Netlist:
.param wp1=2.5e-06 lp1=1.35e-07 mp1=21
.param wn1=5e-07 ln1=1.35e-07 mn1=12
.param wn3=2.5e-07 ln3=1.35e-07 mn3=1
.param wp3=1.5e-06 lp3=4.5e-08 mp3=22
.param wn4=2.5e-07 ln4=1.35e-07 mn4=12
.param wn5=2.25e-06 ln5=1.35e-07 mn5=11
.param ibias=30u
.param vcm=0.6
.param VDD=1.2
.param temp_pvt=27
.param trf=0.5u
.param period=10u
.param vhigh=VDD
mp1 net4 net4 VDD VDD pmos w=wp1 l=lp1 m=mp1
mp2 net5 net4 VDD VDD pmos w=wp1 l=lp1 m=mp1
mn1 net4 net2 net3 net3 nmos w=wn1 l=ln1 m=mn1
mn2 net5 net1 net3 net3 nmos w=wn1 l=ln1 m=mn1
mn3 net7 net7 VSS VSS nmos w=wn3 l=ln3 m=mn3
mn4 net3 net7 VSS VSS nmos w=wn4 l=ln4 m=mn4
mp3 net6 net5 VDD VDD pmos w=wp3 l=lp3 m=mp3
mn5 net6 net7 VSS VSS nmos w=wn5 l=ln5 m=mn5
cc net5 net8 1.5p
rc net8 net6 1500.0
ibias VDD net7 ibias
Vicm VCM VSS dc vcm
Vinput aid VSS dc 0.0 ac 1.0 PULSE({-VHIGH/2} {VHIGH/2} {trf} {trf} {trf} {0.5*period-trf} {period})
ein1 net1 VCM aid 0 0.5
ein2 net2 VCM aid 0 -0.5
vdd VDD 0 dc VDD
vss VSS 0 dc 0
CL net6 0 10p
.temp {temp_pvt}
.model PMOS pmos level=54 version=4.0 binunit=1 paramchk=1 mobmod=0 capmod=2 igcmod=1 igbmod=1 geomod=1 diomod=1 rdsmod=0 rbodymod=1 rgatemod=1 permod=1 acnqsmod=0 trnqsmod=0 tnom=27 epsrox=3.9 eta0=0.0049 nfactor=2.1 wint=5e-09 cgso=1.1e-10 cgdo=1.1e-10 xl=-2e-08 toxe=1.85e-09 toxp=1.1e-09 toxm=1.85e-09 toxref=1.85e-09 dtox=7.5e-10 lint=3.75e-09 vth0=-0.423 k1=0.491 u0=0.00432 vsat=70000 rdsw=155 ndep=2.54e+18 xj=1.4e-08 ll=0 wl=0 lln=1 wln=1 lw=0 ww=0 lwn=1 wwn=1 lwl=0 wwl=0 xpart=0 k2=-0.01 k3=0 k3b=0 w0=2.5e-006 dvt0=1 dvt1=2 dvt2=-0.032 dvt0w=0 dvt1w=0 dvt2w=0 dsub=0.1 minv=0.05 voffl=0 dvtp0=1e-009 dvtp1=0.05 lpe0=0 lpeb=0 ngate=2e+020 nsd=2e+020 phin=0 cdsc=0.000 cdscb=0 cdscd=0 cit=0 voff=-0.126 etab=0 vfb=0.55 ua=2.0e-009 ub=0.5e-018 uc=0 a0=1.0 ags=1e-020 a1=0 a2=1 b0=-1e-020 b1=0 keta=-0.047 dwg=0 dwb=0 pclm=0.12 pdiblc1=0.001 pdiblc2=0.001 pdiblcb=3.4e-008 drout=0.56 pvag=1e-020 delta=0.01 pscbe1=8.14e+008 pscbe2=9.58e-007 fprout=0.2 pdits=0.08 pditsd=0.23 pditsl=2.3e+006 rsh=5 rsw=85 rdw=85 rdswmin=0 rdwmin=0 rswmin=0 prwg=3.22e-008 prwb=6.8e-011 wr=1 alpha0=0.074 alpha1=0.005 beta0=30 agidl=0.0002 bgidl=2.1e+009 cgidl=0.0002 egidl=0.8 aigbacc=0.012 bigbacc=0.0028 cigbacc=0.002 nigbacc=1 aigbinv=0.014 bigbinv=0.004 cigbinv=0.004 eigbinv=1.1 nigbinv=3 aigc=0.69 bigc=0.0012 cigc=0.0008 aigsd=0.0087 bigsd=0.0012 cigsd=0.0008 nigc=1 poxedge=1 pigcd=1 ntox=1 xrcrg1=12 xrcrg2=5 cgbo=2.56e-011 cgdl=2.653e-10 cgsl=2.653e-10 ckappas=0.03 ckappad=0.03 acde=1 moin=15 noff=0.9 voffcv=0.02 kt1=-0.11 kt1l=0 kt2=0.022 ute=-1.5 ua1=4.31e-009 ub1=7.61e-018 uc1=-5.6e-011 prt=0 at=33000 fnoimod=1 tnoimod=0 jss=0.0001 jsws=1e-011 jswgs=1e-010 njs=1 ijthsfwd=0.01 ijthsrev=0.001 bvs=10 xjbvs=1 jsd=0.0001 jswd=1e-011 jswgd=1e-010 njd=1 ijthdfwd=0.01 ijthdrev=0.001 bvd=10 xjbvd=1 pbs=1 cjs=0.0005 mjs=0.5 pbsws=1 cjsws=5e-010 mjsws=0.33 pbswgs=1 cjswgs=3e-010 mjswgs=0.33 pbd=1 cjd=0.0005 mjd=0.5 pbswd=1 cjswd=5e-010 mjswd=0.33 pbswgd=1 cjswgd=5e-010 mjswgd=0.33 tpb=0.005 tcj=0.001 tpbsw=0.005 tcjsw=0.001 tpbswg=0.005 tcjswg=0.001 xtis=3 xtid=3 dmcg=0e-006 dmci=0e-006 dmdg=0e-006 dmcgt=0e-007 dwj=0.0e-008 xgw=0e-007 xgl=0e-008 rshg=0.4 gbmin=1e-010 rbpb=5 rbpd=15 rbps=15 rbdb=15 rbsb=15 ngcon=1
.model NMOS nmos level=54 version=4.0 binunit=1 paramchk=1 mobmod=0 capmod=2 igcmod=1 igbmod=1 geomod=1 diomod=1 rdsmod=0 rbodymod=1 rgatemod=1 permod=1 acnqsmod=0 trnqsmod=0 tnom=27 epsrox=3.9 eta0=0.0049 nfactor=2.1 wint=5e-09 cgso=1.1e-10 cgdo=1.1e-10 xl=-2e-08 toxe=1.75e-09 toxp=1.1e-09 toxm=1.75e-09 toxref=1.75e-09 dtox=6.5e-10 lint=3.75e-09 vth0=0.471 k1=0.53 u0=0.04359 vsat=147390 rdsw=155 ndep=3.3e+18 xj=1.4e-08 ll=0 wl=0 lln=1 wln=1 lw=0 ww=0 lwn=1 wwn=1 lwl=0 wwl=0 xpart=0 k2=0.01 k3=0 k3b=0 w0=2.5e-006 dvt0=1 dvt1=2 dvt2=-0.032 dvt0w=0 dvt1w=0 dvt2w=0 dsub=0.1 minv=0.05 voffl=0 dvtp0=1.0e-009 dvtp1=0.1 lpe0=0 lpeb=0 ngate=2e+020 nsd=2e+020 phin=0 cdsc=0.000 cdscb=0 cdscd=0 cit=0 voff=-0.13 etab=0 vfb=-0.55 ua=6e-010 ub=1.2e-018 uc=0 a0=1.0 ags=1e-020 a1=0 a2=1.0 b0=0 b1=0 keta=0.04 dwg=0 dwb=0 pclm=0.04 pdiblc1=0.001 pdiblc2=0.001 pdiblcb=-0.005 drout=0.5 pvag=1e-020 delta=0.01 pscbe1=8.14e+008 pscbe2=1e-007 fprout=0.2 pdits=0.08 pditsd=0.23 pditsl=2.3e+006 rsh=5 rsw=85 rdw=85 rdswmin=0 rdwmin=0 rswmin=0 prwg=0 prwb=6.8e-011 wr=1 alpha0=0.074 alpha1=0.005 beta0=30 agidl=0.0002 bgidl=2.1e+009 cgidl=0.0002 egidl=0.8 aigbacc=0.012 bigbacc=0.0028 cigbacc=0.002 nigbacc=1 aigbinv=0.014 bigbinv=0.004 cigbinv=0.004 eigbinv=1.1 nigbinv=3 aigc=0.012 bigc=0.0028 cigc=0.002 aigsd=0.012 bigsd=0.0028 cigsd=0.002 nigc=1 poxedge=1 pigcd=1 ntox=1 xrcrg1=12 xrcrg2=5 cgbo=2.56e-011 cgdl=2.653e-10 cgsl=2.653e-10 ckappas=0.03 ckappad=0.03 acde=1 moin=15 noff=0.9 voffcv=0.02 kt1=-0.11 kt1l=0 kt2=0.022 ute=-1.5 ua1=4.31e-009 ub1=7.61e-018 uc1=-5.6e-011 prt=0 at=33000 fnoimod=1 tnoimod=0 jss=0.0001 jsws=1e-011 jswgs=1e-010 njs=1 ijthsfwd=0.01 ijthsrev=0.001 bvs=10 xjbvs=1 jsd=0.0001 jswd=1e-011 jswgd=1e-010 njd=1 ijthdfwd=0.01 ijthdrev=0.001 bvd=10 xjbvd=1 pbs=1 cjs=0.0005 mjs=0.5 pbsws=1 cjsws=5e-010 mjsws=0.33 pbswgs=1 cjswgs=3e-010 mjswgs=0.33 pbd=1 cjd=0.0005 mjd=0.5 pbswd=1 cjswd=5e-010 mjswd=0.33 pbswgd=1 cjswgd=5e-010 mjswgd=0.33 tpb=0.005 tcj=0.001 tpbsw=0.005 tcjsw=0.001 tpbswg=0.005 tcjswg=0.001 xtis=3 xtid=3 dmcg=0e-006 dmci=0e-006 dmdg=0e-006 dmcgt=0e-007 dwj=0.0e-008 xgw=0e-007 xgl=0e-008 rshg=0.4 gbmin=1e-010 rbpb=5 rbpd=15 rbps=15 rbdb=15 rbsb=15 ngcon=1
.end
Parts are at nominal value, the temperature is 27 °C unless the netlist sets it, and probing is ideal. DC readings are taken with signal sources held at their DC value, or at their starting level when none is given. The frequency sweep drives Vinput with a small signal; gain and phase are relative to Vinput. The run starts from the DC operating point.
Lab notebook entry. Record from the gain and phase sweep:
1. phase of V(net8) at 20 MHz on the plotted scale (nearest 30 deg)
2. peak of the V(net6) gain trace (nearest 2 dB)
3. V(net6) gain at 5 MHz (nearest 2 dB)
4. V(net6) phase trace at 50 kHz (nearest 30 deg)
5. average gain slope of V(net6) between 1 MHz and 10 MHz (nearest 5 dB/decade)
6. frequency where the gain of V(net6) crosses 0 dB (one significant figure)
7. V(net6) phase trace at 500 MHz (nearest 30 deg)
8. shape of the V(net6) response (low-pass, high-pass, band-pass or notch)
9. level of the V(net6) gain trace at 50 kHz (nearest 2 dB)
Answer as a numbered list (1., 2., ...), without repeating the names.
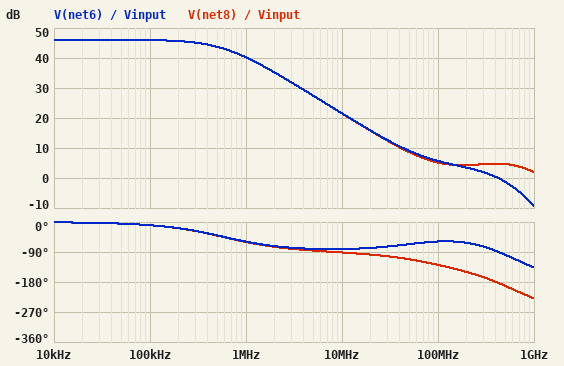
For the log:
1. -90 deg
2. 46 dB
3. 28 dB
4. 0 deg
5. -20 dB/decade
6. 400 MHz
7. -90 deg
8. low-pass
9. 46 dB
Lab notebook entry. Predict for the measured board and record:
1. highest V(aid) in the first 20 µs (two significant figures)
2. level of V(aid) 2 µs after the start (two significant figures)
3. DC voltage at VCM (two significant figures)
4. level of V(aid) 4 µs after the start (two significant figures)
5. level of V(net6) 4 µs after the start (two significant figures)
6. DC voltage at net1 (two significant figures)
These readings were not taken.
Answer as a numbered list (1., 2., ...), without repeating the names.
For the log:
1. 600 mV
2. 600 mV
3. 600 mV
4. 600 mV
5. 1.1 V
6. 600 mV
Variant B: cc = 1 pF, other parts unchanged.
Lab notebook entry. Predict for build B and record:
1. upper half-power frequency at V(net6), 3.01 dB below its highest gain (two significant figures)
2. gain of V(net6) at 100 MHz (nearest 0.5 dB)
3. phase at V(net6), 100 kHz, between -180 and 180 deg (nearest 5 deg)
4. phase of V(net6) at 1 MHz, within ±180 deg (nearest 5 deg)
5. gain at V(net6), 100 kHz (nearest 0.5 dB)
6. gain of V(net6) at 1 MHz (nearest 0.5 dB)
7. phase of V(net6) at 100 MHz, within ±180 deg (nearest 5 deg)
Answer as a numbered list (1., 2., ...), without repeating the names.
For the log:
1. 870 kHz
2. 7.0 dB
3. -5 deg
4. -50 deg
5. 46.0 dB
6. 42.5 dB
7. -70 deg
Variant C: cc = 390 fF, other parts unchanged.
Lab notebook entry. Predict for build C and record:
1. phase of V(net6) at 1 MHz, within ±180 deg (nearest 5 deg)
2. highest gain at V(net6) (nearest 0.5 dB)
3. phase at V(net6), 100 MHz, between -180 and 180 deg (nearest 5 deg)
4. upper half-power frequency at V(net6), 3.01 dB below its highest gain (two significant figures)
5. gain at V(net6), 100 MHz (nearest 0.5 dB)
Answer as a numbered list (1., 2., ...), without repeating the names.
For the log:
1. -25 deg
2. 46.0 dB
3. -95 deg
4. 2.1 MHz
5. 12.5 dB
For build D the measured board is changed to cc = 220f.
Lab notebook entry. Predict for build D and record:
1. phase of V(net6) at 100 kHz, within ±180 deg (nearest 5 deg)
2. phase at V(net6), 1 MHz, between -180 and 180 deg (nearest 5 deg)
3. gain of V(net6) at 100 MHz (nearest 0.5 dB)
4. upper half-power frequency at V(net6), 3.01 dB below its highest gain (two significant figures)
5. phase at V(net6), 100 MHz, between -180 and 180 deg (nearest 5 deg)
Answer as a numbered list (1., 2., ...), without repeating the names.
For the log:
1. 0 deg
2. -15 deg
3. 16.5 dB
4. 3.5 MHz
5. -100 deg
